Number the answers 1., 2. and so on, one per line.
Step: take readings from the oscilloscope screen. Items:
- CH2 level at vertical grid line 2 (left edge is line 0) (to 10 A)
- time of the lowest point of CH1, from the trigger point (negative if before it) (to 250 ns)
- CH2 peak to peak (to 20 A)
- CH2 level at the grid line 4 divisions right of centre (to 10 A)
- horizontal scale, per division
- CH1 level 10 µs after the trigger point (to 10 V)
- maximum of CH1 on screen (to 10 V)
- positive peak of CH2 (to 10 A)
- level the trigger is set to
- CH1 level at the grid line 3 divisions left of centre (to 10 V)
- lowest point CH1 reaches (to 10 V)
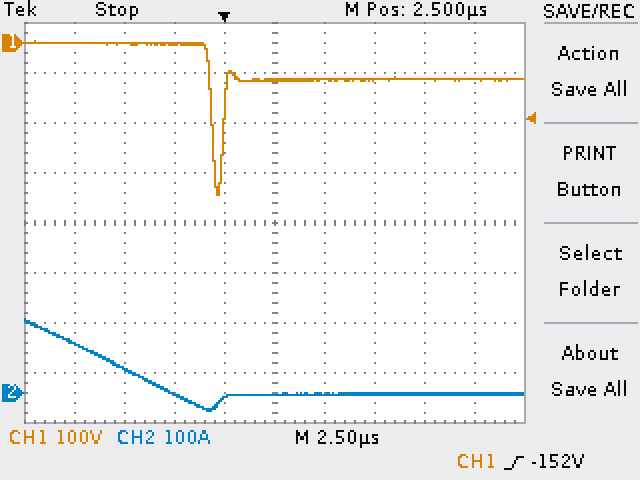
1. 50 A
2. -250 ns
3. 180 A
4. 0 A
5. 2.5 µs
6. -70 V
7. 0 V
8. 150 A
9. -152 V
10. 0 V
11. -300 V
